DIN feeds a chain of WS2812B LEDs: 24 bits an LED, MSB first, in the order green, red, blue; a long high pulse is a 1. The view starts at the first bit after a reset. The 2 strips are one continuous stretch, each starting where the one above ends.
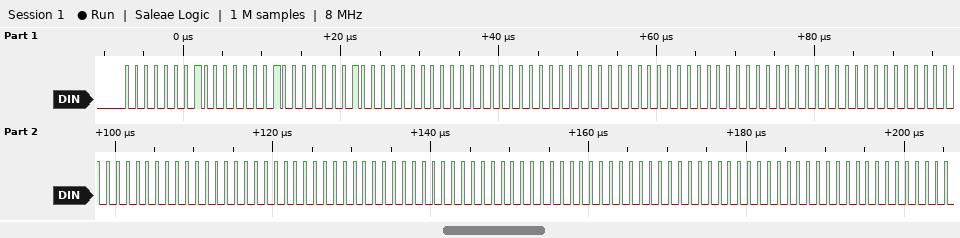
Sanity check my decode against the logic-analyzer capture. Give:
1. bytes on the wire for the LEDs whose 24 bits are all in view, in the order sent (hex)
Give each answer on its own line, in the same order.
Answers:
01 01 01 00 00 00 00 00 00 00 00 00 00 00 00 00 00 00 00 00 00
